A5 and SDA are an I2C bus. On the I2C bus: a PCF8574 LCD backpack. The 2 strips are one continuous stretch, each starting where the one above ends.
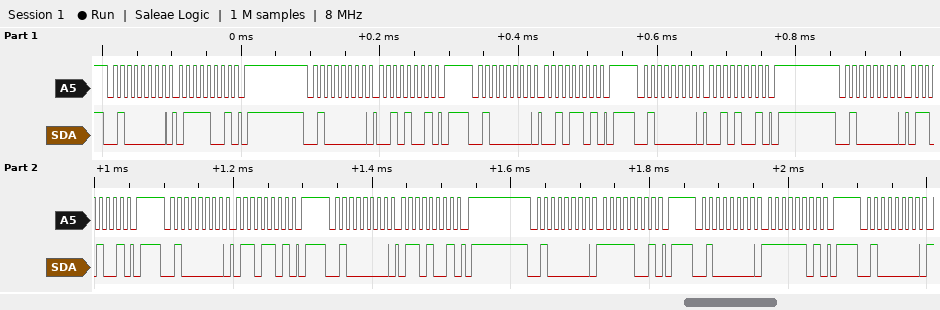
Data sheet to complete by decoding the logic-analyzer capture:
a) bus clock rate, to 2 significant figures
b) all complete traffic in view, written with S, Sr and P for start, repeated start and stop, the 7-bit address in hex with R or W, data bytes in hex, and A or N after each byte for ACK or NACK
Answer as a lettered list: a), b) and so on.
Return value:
a) 100 kHz
b) S 20W A 79 A P S 20W A 29 A P S 20W A 2D A P S 20W A 29 A P S 20W A 69 A P S 20W A 6D A P S 20W A 69 A P S 20W A F9 A P S 20W A FD A P S 20W A
